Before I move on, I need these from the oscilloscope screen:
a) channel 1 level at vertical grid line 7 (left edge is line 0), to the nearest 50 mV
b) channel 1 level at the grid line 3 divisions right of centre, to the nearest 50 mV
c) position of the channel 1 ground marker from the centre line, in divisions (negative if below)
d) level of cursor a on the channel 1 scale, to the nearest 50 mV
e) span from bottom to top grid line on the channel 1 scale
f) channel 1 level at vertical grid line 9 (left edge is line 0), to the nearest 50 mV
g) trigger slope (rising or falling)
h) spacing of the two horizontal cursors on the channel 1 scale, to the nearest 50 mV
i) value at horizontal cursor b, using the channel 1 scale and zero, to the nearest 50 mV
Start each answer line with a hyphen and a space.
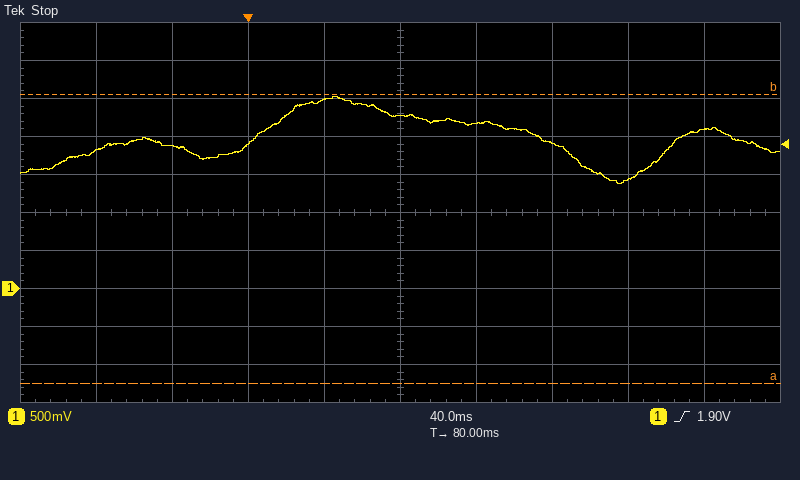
- 1.90 V
- 1.45 V
- -2.0 div
- -1.25 V
- 5 V
- 2.10 V
- rising
- 3.80 V
- 2.55 V
